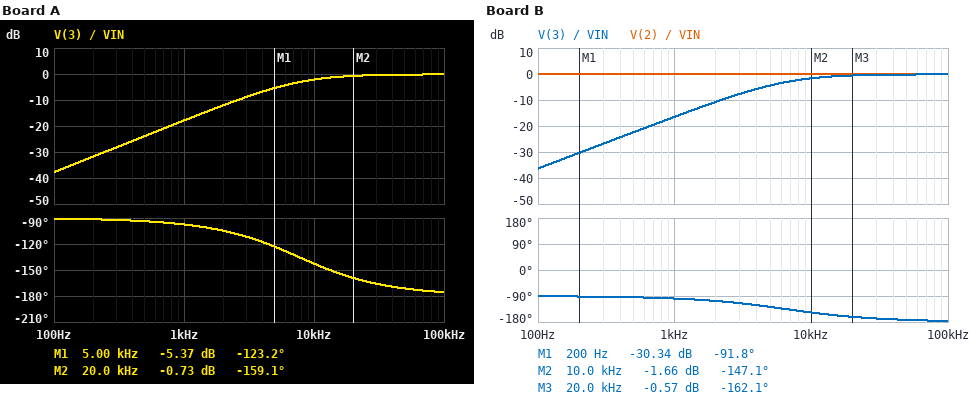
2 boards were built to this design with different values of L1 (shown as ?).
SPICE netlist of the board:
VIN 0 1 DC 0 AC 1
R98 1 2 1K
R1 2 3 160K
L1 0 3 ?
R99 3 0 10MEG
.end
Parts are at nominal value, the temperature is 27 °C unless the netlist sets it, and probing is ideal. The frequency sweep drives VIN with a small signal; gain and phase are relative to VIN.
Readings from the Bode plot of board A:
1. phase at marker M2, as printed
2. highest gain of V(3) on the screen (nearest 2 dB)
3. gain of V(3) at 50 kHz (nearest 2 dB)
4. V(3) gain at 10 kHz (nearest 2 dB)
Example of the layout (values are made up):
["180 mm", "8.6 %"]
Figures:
["-159.1 deg", "0 dB", "0 dB", "-2 dB"]
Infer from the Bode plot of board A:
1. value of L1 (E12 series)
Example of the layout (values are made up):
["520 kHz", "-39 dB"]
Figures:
["3.3 H"]
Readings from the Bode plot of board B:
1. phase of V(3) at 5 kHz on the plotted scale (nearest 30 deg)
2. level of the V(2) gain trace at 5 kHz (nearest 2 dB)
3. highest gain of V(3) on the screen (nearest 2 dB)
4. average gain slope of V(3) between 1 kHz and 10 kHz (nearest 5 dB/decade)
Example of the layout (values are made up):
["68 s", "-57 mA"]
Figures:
["-120 deg", "0 dB", "0 dB", "15 dB/decade"]
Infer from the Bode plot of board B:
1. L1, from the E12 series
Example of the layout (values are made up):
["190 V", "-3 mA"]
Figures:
["3.9 H"]
